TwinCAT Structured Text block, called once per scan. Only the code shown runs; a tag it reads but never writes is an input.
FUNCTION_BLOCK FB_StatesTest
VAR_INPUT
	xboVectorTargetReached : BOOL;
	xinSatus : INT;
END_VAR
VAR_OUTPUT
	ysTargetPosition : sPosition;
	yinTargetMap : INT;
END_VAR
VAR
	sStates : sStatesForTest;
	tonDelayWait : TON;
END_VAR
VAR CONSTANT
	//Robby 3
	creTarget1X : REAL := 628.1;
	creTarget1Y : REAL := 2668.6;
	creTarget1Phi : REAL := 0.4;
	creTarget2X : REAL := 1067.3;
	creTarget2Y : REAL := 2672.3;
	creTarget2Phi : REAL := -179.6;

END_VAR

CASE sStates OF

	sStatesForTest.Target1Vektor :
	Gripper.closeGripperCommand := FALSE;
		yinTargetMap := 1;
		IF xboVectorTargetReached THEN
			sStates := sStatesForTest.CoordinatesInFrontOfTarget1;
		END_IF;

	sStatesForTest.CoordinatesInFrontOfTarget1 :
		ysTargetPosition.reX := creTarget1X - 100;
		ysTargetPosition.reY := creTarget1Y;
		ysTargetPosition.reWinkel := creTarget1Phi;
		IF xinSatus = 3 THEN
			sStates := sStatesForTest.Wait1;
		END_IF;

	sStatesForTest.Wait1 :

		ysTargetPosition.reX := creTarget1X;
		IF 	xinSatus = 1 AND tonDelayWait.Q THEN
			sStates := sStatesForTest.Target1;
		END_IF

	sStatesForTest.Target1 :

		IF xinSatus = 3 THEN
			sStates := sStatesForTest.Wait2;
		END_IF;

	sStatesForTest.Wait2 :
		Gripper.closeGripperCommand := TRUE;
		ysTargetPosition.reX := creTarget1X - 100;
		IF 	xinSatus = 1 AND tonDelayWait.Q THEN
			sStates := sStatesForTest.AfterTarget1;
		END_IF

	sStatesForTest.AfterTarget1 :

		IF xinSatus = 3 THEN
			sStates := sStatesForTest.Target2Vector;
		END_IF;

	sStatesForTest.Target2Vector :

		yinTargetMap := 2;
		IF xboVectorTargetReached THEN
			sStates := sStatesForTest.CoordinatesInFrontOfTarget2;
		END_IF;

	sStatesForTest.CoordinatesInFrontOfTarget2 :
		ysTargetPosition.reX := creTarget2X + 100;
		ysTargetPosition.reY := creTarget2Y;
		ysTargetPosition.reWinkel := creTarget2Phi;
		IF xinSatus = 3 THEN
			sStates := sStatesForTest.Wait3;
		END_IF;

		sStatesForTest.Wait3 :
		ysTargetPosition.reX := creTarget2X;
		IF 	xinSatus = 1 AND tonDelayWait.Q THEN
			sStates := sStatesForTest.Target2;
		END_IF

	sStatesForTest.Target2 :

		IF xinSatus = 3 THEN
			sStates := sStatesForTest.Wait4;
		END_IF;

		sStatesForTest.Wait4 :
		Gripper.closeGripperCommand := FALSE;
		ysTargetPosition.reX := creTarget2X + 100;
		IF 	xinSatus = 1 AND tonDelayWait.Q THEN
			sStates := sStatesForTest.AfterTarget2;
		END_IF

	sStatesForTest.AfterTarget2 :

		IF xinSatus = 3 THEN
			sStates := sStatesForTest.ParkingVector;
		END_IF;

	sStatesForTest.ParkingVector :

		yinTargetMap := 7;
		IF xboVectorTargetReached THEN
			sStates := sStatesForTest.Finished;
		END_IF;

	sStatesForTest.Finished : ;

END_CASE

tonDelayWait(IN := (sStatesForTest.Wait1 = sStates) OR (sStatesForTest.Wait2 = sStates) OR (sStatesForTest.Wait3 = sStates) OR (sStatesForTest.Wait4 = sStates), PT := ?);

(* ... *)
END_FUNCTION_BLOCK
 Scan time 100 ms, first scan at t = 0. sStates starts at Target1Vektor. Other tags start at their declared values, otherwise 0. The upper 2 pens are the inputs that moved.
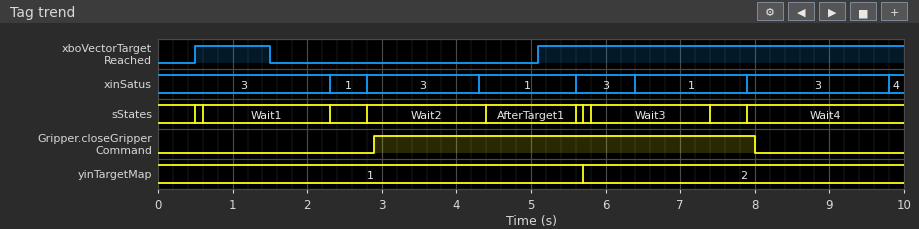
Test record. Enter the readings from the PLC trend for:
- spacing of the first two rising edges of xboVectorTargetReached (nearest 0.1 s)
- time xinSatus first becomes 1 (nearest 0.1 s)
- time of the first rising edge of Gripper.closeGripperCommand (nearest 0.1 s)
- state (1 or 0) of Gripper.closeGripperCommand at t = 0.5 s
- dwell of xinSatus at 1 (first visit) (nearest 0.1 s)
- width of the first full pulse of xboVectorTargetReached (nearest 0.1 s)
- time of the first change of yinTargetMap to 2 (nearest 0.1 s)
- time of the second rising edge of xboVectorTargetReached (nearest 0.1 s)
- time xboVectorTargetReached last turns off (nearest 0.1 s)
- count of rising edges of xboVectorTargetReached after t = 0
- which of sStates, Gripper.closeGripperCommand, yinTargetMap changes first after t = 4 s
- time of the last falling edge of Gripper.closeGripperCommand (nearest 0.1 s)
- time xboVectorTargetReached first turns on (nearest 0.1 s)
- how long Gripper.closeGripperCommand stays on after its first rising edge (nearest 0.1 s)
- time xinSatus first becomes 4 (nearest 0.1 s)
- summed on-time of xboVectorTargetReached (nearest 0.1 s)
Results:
4.6 s
2.3 s
2.9 s
0
0.5 s
1.0 s
5.7 s
5.1 s
1.5 s
2
sStates
8.0 s
0.5 s
5.1 s
9.8 s
5.9 s
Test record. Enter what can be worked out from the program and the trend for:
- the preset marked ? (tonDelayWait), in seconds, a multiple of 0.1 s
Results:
1.5 s
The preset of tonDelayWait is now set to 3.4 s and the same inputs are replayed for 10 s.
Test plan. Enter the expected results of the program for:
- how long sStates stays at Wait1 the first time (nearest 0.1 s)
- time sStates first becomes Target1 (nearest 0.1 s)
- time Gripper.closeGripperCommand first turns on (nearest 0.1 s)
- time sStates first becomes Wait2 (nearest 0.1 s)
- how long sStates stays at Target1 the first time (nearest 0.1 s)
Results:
3.7 s
4.3 s
5.7 s
5.6 s
1.3 s
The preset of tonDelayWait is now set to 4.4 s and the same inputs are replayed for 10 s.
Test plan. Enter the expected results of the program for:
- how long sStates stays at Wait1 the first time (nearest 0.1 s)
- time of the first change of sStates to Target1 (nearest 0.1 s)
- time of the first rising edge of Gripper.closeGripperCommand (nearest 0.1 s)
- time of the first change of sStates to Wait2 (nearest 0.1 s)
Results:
4.5 s
5.1 s
5.7 s
5.6 s
